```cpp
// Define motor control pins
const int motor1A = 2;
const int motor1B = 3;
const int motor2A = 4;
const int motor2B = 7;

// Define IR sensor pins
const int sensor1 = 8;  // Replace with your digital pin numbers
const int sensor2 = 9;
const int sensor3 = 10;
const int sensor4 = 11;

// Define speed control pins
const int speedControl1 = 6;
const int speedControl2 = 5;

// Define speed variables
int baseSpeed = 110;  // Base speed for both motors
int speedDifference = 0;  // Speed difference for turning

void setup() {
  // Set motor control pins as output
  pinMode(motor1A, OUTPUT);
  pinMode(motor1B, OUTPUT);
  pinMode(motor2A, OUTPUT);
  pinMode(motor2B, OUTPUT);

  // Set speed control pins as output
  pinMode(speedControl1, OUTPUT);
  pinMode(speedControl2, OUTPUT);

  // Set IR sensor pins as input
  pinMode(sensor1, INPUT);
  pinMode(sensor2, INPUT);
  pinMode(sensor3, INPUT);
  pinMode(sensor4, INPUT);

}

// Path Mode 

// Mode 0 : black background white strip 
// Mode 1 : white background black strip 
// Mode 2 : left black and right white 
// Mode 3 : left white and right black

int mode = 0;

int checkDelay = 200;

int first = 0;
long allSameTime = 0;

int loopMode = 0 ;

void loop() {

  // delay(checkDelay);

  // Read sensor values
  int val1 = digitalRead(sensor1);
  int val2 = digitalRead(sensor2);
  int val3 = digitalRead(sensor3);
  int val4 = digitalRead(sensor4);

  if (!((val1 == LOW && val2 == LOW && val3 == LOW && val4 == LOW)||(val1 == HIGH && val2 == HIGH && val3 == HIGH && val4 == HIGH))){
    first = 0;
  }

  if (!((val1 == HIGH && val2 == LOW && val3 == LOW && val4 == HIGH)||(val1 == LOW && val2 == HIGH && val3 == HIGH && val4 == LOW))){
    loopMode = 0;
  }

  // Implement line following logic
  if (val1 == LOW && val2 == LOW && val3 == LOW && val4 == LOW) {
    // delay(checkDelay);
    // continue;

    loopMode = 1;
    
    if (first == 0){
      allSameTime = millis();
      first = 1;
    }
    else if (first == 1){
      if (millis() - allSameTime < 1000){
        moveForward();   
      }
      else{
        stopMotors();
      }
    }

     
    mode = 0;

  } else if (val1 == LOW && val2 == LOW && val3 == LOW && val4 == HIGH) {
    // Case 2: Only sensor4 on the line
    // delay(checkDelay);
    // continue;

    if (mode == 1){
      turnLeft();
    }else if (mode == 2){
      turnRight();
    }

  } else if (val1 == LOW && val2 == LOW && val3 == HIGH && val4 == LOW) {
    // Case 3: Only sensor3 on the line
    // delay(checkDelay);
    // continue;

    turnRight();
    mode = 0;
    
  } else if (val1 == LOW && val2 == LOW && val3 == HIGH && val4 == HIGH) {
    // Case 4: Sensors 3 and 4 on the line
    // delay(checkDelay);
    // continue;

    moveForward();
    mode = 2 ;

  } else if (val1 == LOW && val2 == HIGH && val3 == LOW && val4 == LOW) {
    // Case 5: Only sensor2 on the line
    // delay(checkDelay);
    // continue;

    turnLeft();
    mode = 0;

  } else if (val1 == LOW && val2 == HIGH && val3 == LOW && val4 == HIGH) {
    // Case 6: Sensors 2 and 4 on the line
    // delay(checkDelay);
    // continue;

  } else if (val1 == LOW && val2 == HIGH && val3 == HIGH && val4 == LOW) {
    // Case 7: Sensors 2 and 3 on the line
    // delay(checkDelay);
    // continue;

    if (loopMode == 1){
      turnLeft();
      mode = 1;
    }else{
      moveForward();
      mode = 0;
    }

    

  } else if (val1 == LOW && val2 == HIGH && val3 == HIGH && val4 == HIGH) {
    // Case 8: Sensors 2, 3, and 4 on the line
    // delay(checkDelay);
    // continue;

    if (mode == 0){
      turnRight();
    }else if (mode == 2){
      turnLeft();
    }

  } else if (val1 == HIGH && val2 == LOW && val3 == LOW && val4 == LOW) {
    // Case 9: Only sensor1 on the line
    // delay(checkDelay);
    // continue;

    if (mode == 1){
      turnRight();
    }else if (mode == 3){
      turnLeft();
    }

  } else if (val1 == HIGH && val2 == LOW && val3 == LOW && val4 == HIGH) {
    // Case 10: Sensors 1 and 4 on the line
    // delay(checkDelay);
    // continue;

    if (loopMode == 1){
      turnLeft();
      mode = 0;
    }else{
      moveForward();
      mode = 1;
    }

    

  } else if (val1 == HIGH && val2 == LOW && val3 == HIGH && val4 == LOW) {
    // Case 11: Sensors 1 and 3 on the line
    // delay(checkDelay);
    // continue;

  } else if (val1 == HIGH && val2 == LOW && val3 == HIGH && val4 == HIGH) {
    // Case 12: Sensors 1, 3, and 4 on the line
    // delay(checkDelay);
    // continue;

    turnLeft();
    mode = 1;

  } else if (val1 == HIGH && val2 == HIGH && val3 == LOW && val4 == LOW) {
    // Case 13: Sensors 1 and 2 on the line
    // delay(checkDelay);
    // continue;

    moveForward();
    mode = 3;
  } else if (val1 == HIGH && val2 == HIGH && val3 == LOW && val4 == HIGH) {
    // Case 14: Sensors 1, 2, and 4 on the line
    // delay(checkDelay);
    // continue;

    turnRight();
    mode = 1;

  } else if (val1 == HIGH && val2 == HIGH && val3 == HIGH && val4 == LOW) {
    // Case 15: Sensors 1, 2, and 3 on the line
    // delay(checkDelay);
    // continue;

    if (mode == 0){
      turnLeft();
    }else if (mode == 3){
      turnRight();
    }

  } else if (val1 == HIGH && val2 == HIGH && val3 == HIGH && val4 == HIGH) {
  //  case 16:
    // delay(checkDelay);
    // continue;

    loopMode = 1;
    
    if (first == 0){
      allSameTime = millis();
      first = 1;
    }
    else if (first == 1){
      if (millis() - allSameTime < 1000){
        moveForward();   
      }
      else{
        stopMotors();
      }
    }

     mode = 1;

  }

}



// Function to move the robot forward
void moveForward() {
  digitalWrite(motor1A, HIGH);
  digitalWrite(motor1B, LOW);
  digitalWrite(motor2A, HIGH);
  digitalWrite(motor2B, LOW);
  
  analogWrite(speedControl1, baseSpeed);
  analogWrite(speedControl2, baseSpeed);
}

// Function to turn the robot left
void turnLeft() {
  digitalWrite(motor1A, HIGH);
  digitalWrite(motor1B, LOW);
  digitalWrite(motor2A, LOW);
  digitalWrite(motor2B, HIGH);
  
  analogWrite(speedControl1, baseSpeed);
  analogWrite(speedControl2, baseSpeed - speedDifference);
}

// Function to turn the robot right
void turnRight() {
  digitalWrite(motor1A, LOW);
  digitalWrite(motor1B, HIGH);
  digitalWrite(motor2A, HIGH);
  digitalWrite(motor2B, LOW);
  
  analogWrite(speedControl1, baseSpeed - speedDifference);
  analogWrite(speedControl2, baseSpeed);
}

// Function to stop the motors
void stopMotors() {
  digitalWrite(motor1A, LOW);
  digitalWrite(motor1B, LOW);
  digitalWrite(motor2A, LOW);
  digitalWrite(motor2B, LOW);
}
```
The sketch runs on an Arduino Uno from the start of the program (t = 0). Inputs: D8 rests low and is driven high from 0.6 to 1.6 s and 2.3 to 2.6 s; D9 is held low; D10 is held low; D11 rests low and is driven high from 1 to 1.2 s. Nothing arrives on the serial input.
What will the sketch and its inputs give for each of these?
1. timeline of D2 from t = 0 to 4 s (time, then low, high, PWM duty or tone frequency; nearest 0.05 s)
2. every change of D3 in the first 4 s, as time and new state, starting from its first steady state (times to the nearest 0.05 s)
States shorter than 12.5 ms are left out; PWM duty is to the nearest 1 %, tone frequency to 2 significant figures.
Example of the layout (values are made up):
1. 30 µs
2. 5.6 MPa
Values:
1. 0 s high; 1.2 s low; 1.6 s high; 3.6 s low
2. 0 s low; 1.2 s high; 1.6 s low
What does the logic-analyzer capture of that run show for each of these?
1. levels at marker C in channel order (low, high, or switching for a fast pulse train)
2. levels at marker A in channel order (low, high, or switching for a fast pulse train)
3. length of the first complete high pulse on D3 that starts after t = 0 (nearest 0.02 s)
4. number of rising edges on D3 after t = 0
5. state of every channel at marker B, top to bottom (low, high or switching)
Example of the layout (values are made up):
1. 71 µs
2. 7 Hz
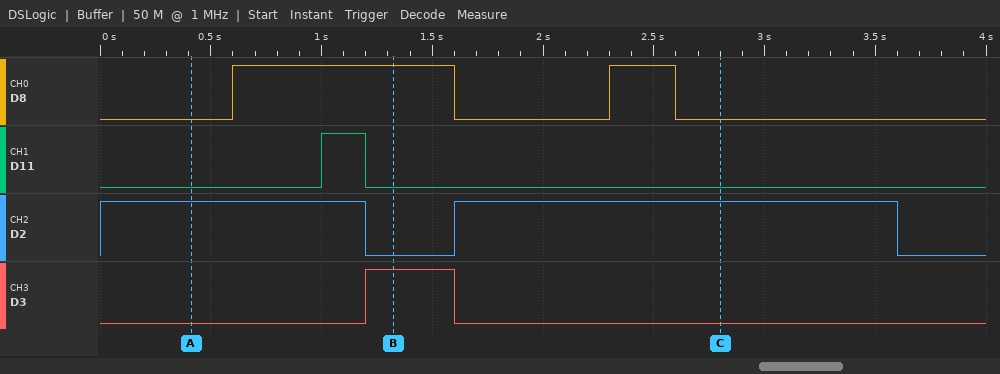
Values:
1. D8 low, D11 low, D2 high, D3 low
2. D8 low, D11 low, D2 high, D3 low
3. 0.40 s
4. 1
5. D8 high, D11 low, D2 low, D3 high
